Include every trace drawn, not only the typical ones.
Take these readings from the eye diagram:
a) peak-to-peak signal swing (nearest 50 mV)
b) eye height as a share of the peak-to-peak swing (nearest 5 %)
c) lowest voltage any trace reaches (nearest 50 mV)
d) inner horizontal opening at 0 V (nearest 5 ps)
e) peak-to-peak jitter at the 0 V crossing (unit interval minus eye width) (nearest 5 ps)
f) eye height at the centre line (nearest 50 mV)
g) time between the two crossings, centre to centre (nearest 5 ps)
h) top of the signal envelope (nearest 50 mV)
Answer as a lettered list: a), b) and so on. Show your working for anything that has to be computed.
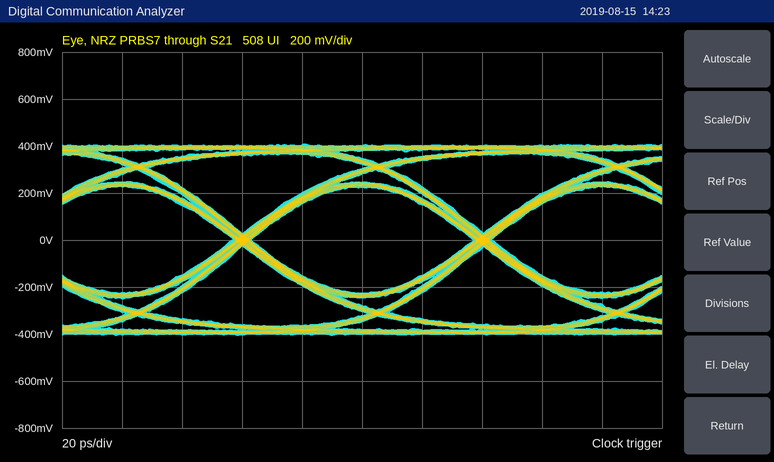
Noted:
a) 800 mV
b) 450 mV / 800 mV ≈ 56.2 %, so 55 % to the nearest 5 %
c) -400 mV
d) 75 ps
e) 5 ps
f) 450 mV
g) 80 ps
h) 400 mV
